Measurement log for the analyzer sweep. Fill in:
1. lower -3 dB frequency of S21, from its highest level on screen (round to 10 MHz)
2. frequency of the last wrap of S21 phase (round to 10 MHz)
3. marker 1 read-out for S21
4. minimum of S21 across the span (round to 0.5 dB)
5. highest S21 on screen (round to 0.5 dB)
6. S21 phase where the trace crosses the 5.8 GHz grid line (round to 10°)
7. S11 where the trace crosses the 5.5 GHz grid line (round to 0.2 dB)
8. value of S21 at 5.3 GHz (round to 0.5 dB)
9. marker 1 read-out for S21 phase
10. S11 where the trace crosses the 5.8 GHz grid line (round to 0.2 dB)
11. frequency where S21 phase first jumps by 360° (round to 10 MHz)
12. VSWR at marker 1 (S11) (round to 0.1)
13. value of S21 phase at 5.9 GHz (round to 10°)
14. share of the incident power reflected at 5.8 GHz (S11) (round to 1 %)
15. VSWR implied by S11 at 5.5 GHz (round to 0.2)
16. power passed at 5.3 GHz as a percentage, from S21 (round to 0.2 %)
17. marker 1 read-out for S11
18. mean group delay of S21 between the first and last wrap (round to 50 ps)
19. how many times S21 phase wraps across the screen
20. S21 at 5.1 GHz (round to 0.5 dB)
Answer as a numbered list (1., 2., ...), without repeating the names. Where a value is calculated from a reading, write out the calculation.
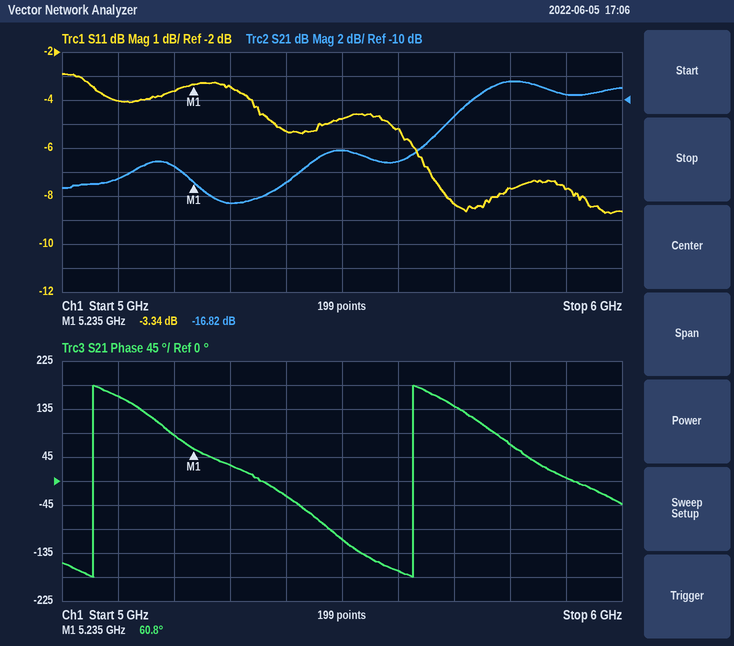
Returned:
1. 5.70 GHz
2. 5.63 GHz
3. -16.82 dB
4. -18.5 dB
5. -8.5 dB
6. 70°
7. -4.8 dB
8. -18.5 dB
9. 60.8°
10. -7.6 dB
11. 5.06 GHz
12. (1 + 0.6808)/(1 − 0.6808) ≈ 5.3
13. 10°
14. 10^(-7.6/10) ≈ 17 %
15. |Γ| = 10^(-4.8/20) = 0.5754; VSWR = (1 + 0.5754)/(1 − 0.5754) ≈ 3.71, so 3.8 to the nearest 0.2
16. 10^(-18.5/10) ≈ 1.4 %
17. -3.34 dB
18. 1 cycle / (5.63 GHz − 5.06 GHz) ≈ 1.75 ns
19. 2
20. -16.5 dB
